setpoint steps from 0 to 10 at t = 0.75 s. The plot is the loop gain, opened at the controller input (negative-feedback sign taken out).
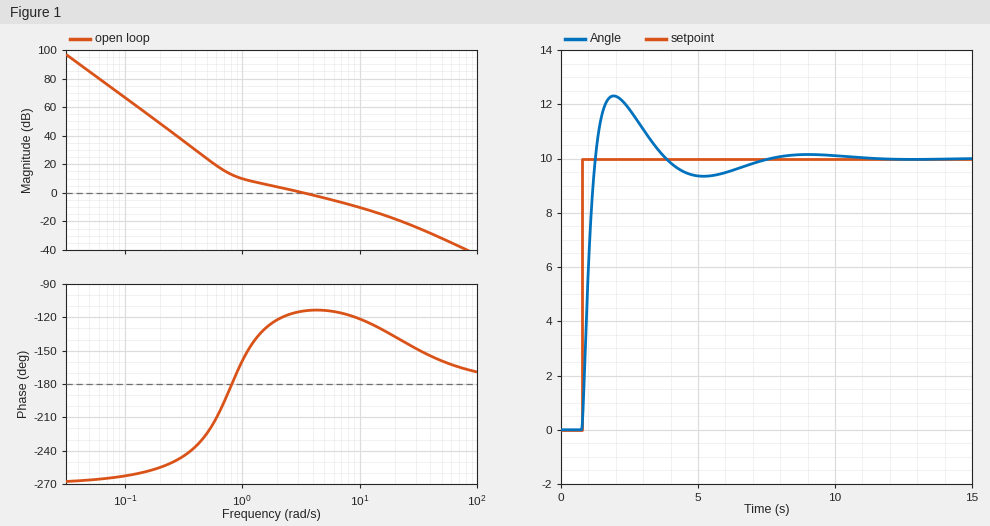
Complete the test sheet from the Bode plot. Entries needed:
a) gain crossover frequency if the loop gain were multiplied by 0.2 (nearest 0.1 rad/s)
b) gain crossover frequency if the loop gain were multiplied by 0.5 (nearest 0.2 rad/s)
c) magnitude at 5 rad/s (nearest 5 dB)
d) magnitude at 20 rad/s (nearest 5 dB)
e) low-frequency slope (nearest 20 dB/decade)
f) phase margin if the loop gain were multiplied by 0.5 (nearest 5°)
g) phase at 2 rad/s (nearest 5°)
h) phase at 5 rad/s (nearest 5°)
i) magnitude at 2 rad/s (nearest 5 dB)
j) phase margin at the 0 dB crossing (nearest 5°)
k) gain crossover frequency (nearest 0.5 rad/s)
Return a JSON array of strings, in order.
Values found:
["0.8 rad/s", "1.6 rad/s", "-5 dB", "-20 dB", "-60 dB/decade", "50°", "-120°", "-115°", "5 dB", "65°", "3.5 rad/s"]
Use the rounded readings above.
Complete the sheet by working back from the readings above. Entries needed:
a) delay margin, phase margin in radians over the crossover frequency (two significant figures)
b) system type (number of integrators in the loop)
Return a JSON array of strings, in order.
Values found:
["0.32 s", "3"]
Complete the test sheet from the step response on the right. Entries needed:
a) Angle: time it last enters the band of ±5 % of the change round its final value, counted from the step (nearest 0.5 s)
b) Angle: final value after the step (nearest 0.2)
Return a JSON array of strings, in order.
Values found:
["5.5 s", "10.0"]
